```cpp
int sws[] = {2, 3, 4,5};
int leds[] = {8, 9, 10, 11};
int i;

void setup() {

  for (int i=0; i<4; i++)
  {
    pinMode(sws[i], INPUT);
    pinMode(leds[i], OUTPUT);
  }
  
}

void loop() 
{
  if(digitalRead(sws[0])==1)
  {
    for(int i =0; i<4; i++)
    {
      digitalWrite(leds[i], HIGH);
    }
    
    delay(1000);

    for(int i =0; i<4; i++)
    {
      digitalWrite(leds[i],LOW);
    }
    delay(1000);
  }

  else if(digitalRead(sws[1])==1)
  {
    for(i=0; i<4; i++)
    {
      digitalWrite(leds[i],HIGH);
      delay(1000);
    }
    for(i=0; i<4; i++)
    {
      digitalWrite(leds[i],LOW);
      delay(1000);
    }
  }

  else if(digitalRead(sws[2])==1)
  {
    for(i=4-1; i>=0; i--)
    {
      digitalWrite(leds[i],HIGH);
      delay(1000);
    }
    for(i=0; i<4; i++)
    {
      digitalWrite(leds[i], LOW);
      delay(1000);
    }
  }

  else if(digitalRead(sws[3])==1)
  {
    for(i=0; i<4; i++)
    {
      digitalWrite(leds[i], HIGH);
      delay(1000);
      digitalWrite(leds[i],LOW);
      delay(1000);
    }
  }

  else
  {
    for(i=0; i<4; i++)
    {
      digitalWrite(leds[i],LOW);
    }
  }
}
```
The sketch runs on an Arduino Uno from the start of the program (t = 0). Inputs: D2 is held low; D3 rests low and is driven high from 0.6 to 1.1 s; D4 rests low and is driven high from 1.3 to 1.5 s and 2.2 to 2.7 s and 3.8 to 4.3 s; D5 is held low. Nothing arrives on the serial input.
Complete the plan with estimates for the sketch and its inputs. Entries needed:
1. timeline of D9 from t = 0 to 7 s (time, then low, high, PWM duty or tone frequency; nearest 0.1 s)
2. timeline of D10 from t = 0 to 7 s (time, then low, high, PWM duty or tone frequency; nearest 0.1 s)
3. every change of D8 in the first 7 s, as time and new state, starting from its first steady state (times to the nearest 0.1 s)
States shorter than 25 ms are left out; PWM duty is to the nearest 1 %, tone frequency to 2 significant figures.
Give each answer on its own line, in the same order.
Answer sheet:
0 s low; 1.6 s high; 5.6 s low
0 s low; 2.6 s high; 6.6 s low
0 s low; 0.6 s high; 4.6 s low
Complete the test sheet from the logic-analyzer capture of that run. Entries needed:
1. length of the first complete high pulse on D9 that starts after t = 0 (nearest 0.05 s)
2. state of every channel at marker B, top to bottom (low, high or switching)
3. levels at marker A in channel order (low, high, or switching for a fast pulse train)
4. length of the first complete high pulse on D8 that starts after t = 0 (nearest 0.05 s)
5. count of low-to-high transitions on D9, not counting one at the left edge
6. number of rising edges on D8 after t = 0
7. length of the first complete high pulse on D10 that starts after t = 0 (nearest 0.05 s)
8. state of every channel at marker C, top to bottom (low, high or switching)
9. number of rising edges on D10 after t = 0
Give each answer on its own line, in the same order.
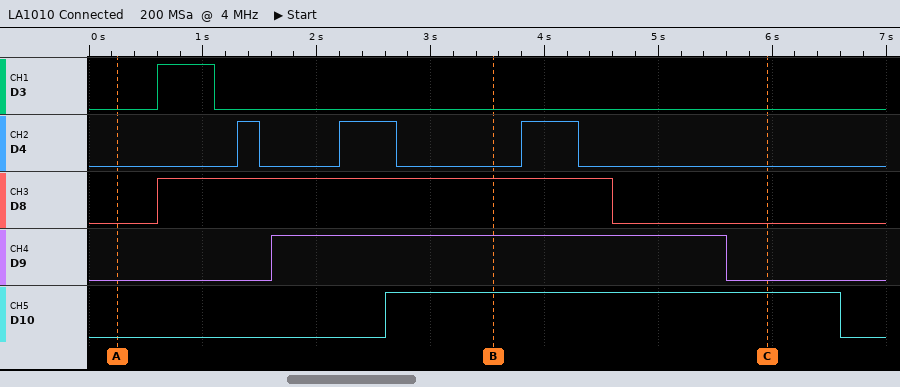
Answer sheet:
4.00 s
D3 low, D4 low, D8 high, D9 high, D10 high
D3 low, D4 low, D8 low, D9 low, D10 low
4.00 s
1
1
4.00 s
D3 low, D4 low, D8 low, D9 low, D10 high
1
